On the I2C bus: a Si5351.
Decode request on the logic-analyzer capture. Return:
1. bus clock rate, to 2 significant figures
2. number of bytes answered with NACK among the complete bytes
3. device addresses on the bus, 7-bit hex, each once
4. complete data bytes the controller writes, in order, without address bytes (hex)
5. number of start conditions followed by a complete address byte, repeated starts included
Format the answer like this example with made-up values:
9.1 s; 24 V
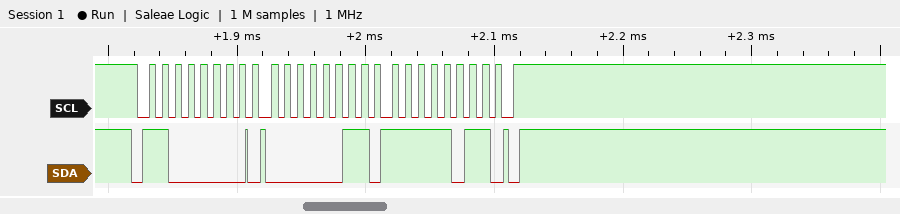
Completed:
100 kHz; 0; 0x60; 03 FB; 1
